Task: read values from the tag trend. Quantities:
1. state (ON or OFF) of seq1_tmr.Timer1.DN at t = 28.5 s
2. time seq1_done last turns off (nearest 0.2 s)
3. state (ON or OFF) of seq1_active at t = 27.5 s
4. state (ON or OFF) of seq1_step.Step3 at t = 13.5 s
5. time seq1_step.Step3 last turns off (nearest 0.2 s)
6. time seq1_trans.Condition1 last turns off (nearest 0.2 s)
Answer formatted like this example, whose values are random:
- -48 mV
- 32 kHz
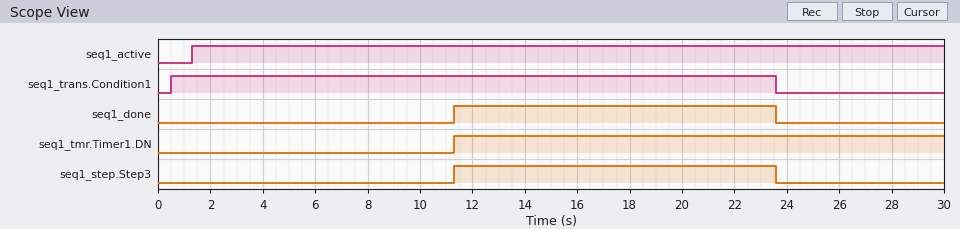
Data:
- ON
- 23.6 s
- ON
- ON
- 23.6 s
- 23.6 s
